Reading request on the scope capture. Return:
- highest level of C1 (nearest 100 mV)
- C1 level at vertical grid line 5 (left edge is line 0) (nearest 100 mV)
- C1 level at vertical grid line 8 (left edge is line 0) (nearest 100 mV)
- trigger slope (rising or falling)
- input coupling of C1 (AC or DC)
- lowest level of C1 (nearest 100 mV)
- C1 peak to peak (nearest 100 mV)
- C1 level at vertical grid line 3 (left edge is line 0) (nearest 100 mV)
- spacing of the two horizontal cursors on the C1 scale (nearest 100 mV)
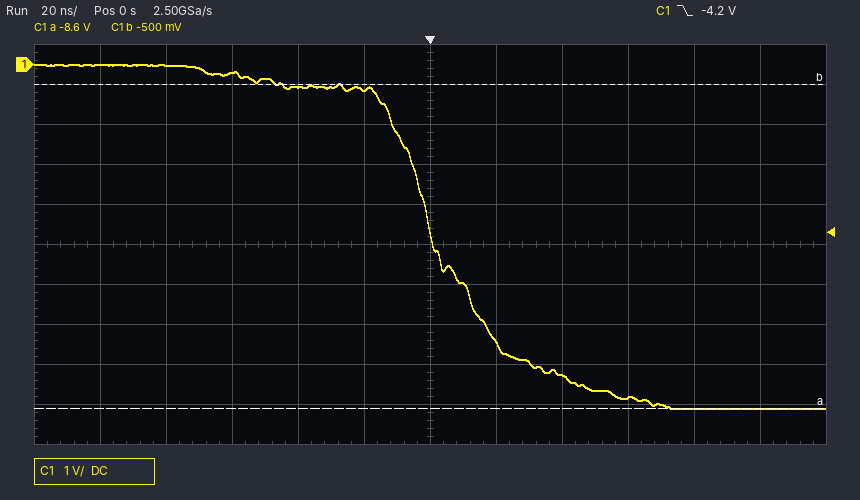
0.0 V
-600 mV
-7.8 V
falling
DC
-8.6 V
8.6 V
-200 mV
8.1 V
